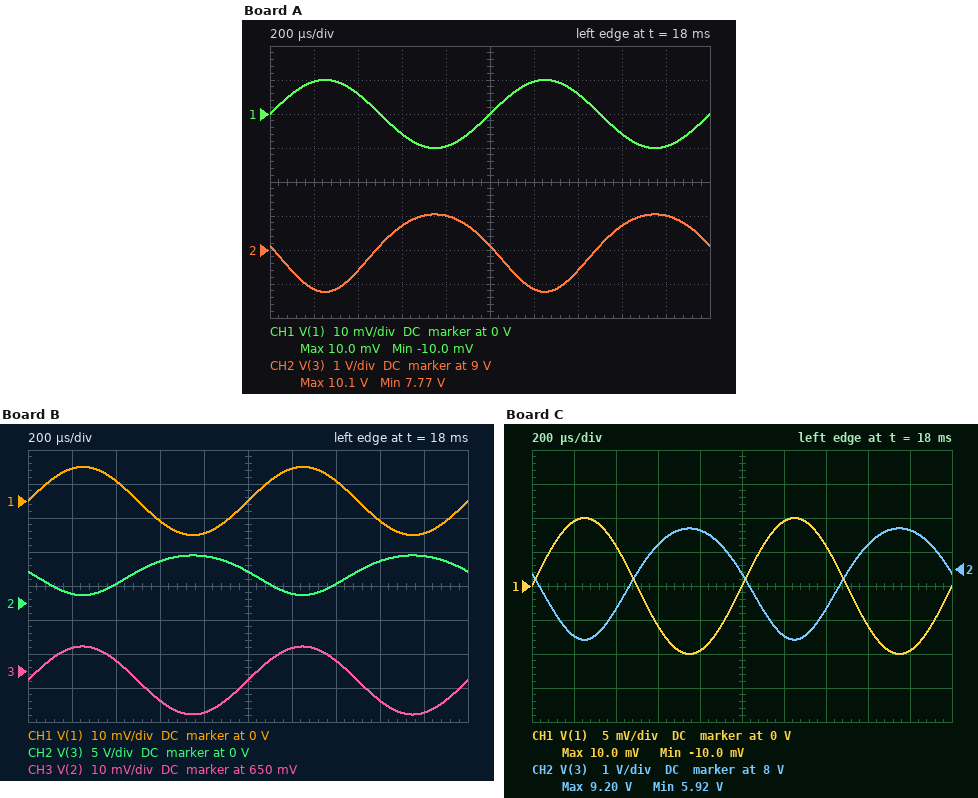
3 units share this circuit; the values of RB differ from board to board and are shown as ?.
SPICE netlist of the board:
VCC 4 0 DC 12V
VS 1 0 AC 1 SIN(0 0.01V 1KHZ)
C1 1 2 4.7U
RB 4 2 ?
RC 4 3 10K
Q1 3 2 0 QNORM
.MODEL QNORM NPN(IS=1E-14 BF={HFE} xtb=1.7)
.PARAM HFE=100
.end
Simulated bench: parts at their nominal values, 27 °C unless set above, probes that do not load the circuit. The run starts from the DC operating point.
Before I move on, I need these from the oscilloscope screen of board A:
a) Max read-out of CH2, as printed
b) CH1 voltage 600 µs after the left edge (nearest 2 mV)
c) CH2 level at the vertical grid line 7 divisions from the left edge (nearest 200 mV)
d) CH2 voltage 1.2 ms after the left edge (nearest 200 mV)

10.1 V
-6 mV
8.4 V
7.8 V
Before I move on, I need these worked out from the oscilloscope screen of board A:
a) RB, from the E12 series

3.9 MΩ
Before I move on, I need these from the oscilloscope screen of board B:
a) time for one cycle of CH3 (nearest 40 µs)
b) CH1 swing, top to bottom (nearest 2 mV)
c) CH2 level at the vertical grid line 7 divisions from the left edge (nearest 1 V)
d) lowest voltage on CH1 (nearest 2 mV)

1.00 ms
20 mV
3 V
-10 mV
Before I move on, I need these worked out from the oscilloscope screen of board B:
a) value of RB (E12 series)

1.5 MΩ
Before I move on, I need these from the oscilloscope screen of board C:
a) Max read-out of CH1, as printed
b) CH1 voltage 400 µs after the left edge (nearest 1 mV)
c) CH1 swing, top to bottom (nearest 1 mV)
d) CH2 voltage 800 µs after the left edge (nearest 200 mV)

10.0 mV
6 mV
20 mV
9.2 V
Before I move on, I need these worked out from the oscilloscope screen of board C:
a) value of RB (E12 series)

2.7 MΩ
